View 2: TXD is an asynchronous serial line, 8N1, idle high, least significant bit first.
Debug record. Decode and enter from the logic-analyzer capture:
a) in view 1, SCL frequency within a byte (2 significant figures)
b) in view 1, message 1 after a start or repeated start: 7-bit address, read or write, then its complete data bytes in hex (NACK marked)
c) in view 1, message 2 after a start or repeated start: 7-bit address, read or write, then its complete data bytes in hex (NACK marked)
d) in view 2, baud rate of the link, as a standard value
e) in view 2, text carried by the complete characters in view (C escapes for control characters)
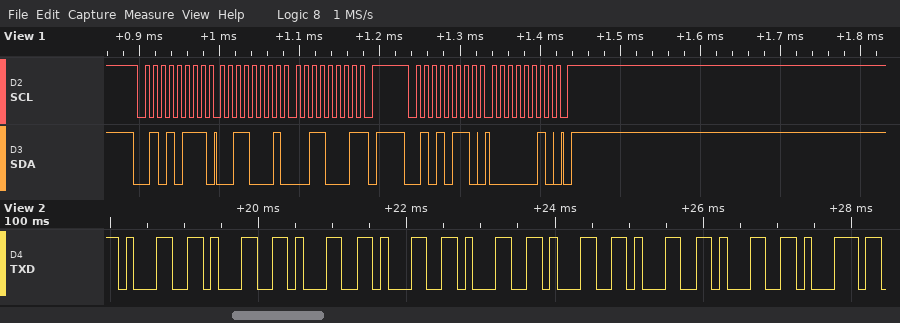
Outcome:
100 kHz
0x2B read: 31 31 NACK
0x2B write: 02
9600 baud
"11111111q"
